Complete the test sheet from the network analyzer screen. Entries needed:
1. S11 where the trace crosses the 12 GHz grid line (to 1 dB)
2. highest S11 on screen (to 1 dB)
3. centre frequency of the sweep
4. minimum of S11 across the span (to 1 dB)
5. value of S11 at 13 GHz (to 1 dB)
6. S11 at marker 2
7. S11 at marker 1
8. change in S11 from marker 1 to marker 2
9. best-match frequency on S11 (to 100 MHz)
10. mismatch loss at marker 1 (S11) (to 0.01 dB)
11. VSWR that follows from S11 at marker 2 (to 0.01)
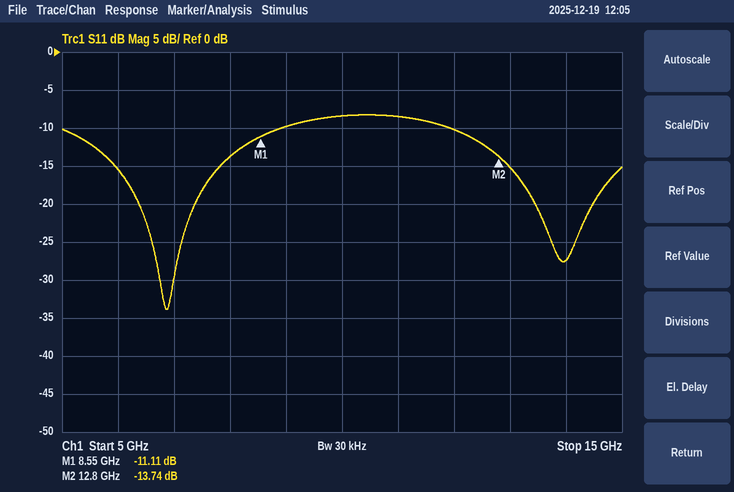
-10 dB
-8 dB
10 GHz
-34 dB
-15 dB
-13.74 dB
-11.11 dB
-2.63 dB
6.9 GHz
0.35 dB
1.52
